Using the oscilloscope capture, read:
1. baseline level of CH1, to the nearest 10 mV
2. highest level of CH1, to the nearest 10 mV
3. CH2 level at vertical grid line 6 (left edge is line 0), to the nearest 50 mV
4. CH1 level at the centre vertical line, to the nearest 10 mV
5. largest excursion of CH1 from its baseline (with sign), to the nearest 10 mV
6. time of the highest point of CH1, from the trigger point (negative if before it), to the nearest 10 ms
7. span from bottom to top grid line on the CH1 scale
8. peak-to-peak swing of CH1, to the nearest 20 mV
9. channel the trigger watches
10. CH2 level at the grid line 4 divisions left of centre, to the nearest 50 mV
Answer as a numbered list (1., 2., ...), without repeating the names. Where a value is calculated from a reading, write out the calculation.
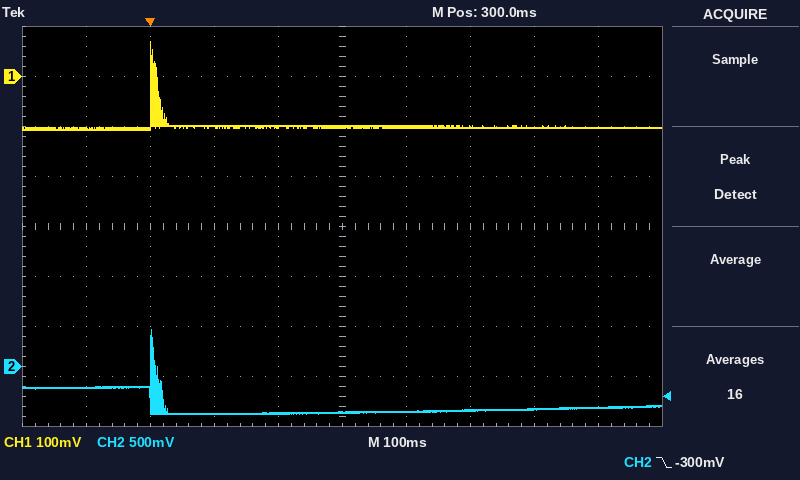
1. -100 mV
2. 70 mV
3. -450 mV
4. -100 mV
5. 70 mV − (-100 mV) = +170 mV
6. 0 ms
7. 800 mV
8. 180 mV
9. CH2
10. -200 mV
